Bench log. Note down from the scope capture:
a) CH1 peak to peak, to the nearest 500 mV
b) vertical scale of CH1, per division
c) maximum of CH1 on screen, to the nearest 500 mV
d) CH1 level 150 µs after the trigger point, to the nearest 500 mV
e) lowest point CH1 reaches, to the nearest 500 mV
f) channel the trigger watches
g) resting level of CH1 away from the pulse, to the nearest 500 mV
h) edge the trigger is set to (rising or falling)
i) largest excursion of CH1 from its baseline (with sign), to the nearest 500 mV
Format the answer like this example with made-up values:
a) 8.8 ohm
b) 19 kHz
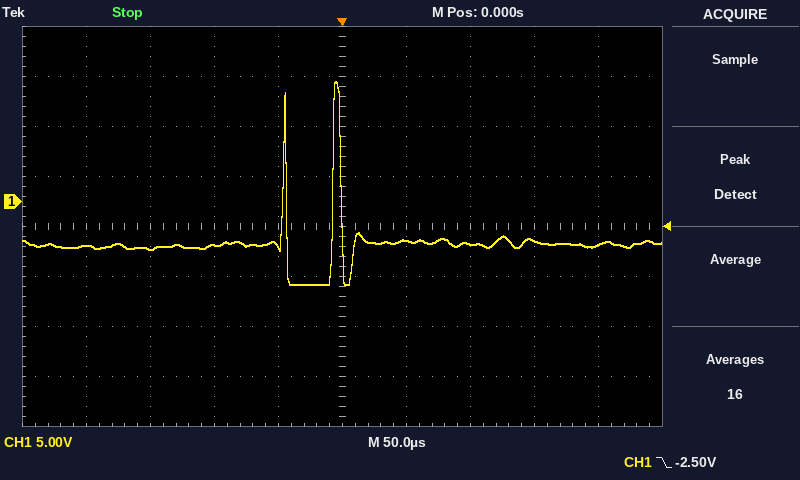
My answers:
a) 20.5 V
b) 5 V
c) 12.0 V
d) -4.0 V
e) -8.5 V
f) CH1
g) -4.5 V
h) falling
i) +16.5 V
